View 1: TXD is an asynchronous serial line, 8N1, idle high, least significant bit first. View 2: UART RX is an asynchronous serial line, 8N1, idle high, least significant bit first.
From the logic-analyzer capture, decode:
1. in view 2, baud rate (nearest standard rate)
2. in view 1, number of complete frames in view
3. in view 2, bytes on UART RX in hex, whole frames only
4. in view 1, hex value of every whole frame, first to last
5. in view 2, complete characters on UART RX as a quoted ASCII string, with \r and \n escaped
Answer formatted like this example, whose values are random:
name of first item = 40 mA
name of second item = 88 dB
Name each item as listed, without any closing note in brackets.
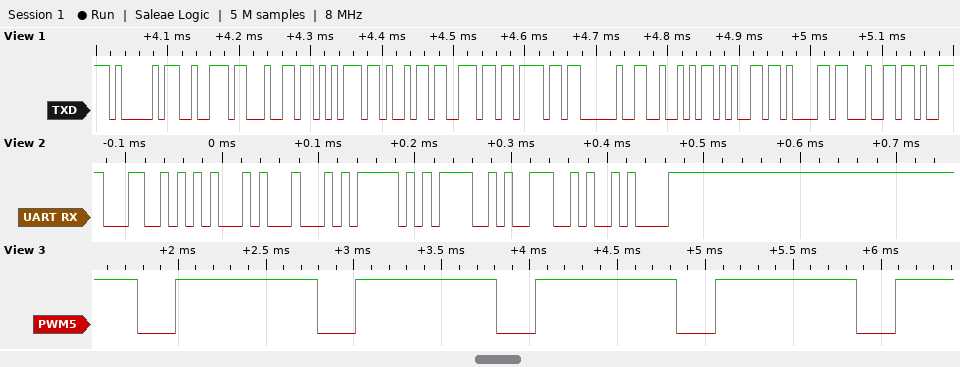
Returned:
in view 2, baud rate = 115200 baud
in view 1, number of complete frames in view = 12
in view 2, bytes on UART RX in hex, whole frames only = 4C 45 44 5F 4F 4E 0A
in view 1, hex value of every whole frame, first to last = 0x41 0x72 0x64 0x75 0x69 0x6E 0x6F 0x20 0x52 0x65 0x61 0x64
in view 2, complete characters on UART RX as a quoted ASCII string, with \r and \n escaped = "LED_ON\n"
